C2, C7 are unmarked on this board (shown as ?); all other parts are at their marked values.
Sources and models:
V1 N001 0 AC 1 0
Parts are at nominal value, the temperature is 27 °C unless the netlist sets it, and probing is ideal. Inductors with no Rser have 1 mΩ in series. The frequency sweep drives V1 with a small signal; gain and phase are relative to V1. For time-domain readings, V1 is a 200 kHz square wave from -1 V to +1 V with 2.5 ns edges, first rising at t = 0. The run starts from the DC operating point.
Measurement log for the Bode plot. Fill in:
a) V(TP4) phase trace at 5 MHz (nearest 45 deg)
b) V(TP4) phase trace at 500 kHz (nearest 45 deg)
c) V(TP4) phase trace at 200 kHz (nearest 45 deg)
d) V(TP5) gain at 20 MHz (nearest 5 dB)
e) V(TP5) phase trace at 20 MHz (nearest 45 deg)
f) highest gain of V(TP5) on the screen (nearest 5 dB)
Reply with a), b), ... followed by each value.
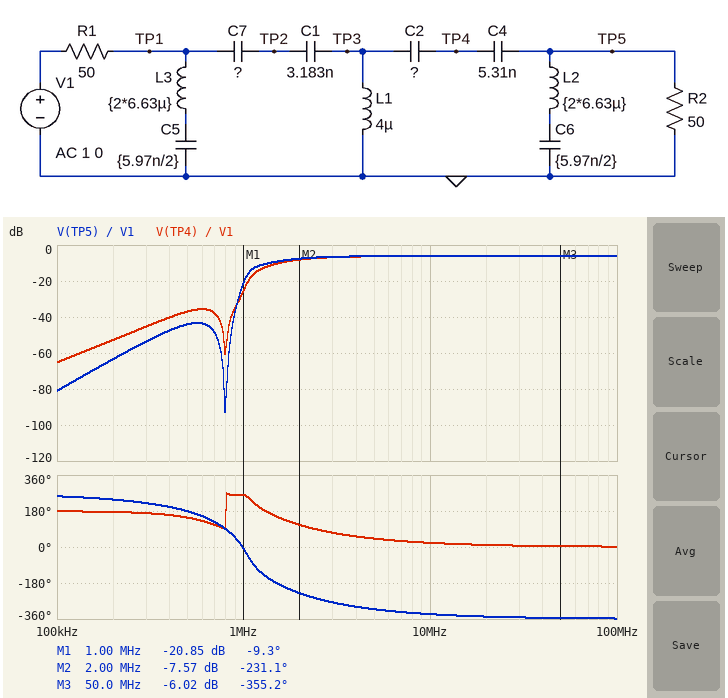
a) 45 deg
b) 135 deg
c) 180 deg
d) -5 dB
e) -360 deg
f) -5 dB
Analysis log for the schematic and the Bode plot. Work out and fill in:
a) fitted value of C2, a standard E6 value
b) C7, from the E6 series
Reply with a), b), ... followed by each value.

a) 1 nF
b) 6.8 nF
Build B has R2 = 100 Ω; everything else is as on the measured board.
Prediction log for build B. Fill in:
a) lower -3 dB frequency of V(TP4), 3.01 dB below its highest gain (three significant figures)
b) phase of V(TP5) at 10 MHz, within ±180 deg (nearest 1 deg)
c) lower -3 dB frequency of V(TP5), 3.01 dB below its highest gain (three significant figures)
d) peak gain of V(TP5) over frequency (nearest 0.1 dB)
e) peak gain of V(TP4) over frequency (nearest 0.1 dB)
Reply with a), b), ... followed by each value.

a) 1.48 MHz
b) 22 deg
c) 1.28 MHz
d) -3.4 dB
e) -3.5 dB
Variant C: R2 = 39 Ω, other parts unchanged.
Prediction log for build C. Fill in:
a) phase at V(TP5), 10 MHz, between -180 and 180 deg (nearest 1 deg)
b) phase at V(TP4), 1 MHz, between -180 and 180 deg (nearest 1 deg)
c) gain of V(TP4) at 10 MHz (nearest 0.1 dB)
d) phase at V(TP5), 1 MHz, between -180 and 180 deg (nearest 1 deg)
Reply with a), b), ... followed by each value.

a) 25 deg
b) -106 deg
c) -7.2 dB
d) -16 deg
